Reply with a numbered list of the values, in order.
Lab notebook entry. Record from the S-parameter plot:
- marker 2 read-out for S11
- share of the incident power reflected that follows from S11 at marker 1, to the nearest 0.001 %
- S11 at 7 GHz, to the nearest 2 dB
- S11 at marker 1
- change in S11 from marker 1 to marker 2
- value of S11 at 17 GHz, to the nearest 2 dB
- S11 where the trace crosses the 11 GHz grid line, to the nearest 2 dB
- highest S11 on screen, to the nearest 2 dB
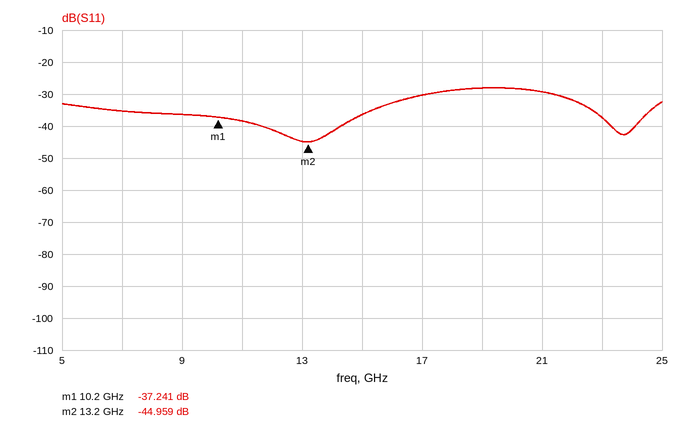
1. -44.959 dB
2. 0.019 %
3. -36 dB
4. -37.241 dB
5. -7.718 dB
6. -30 dB
7. -38 dB
8. -28 dB
